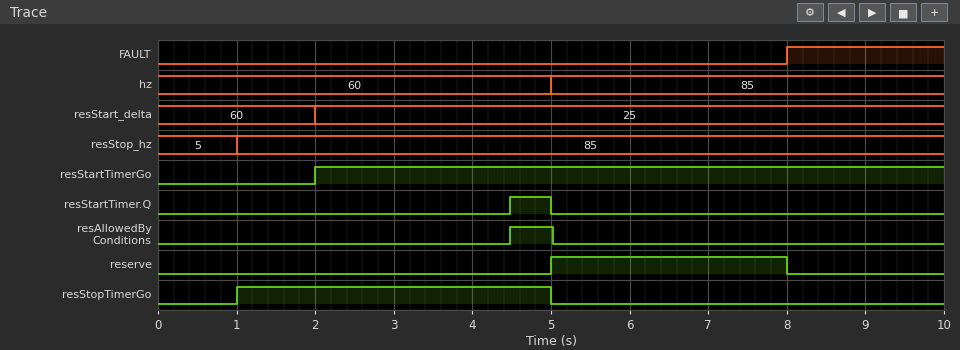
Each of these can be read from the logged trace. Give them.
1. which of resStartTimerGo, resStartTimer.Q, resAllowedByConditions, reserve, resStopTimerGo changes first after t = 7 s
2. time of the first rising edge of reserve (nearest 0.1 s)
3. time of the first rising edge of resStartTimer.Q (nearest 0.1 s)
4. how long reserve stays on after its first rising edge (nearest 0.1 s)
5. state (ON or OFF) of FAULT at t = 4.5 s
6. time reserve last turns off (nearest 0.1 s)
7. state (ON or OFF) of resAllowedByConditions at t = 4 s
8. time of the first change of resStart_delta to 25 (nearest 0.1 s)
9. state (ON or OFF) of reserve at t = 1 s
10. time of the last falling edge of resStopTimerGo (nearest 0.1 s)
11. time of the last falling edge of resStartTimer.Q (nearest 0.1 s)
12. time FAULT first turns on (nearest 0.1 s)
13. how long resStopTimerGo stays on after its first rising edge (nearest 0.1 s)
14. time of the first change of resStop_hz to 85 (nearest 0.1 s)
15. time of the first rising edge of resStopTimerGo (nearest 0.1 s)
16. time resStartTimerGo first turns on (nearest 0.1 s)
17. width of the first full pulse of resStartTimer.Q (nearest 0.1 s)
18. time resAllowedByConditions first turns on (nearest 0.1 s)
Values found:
reserve
5.0 s
4.5 s
3.0 s
OFF
8.0 s
OFF
2.0 s
OFF
5.0 s
5.0 s
8.0 s
4.0 s
1.0 s
1.0 s
2.0 s
0.5 s
4.5 s
